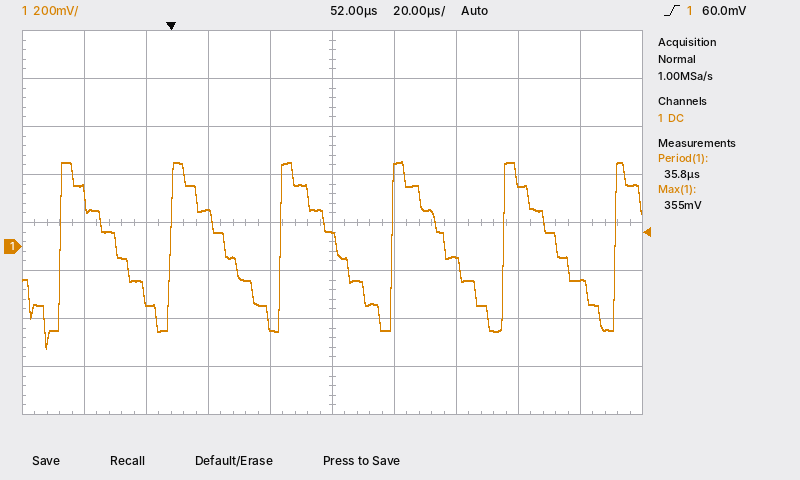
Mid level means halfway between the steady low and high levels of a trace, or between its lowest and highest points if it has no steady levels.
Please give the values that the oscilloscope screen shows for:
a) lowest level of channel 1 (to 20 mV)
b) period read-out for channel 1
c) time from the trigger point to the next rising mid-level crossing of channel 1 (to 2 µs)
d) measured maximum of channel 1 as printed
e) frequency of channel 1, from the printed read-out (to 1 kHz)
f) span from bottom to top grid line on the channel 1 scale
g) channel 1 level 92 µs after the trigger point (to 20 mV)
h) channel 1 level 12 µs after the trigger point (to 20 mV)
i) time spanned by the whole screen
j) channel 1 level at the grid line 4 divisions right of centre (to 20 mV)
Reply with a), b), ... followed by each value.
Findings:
a) -420 mV
b) 35.8 µs
c) 36 µs
d) 355 mV
e) 28 kHz
f) 1.6 V
g) -60 mV
h) 140 mV
i) 200 µs
j) -140 mV
